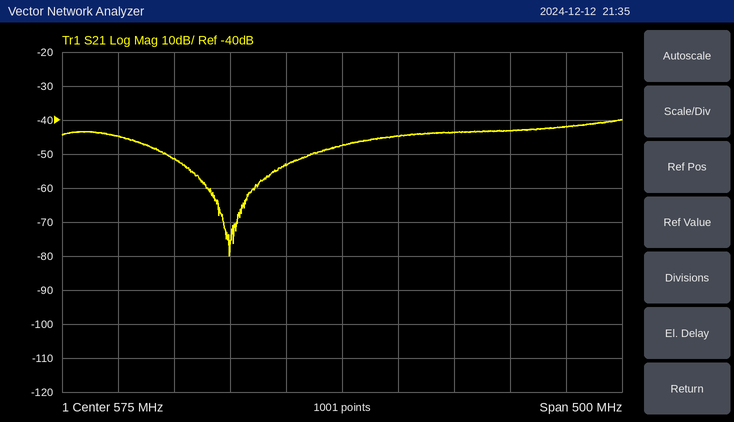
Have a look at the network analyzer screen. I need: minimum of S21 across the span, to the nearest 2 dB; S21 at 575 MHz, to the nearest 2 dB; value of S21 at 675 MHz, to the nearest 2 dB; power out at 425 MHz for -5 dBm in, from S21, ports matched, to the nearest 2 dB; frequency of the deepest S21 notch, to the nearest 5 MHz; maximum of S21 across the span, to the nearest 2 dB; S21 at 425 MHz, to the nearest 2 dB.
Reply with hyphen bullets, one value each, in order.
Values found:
- -80 dB
- -48 dB
- -44 dB
- -56 dBm
- 475 MHz
- -40 dB
- -52 dB
